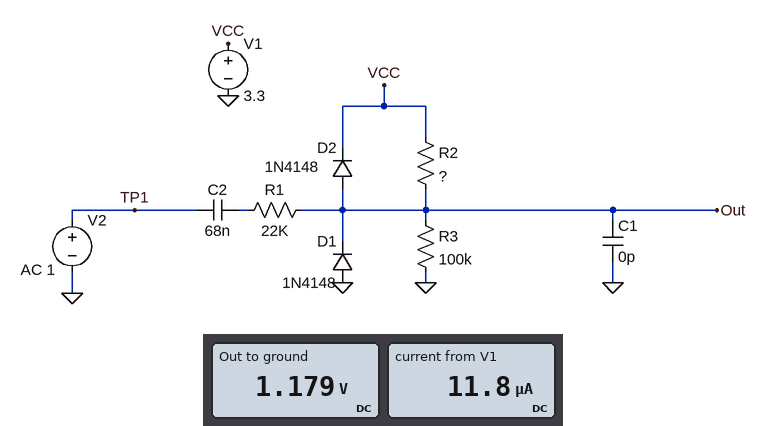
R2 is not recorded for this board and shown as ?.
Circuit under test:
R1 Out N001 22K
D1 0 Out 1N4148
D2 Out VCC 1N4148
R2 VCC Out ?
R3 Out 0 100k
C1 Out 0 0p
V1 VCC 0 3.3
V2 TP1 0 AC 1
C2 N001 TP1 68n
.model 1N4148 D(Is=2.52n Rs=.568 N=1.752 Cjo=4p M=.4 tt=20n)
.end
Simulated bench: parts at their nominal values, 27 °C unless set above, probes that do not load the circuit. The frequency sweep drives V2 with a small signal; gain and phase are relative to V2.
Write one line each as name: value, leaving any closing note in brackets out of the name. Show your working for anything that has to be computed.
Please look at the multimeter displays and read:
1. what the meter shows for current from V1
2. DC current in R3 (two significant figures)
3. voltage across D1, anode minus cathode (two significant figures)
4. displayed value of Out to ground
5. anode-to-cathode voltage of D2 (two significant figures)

what the meter shows for current from V1: 11.8 µA
DC current in R3: (1.179 V) / 100 kΩ = 12 µA
voltage across D1, anode minus cathode: 0 V - 1.179 V = -1.2 V
displayed value of Out to ground: 1.179 V
anode-to-cathode voltage of D2: 1.179 V - 3.3 V = -2.1 V
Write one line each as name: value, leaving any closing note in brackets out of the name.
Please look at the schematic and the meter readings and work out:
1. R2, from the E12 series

R2, from the E12 series: 180 kΩ
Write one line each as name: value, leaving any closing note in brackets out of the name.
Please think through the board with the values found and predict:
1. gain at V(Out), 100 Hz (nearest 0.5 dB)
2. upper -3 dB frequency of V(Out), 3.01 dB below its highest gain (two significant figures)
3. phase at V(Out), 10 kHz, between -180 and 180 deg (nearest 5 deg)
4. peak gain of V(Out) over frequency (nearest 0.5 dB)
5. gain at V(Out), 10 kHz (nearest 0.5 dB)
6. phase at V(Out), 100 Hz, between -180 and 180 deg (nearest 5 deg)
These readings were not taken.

gain at V(Out), 100 Hz: -3.0 dB
upper -3 dB frequency of V(Out), 3.01 dB below its highest gain: 1.8 MHz
phase at V(Out), 10 kHz, between -180 and 180 deg: 0 deg
peak gain of V(Out) over frequency: -2.5 dB
gain at V(Out), 10 kHz: -2.5 dB
phase at V(Out), 100 Hz, between -180 and 180 deg: 15 deg
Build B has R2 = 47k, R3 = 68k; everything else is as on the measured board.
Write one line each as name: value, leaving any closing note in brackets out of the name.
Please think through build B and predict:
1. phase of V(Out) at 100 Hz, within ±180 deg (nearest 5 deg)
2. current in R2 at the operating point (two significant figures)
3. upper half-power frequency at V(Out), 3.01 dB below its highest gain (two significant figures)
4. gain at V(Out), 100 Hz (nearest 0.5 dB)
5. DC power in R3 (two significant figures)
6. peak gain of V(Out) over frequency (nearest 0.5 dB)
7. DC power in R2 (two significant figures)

phase of V(Out) at 100 Hz, within ±180 deg: 25 deg
current in R2 at the operating point: 29 µA
upper half-power frequency at V(Out), 3.01 dB below its highest gain: 2.4 MHz
gain at V(Out), 100 Hz: -6.0 dB
DC power in R3: 56 µW
peak gain of V(Out) over frequency: -5.0 dB
DC power in R2: 39 µW
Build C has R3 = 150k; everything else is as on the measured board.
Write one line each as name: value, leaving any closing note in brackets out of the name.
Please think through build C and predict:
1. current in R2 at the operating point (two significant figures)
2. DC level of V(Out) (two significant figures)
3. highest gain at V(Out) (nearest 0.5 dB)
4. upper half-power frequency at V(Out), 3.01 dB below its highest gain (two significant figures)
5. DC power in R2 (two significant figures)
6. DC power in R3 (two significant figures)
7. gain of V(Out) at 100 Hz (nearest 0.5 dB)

current in R2 at the operating point: 10 µA
DC level of V(Out): 1.5 V
highest gain at V(Out): -2.0 dB
upper half-power frequency at V(Out), 3.01 dB below its highest gain: 1.7 MHz
DC power in R2: 18 µW
DC power in R3: 15 µW
gain of V(Out) at 100 Hz: -2.5 dB
